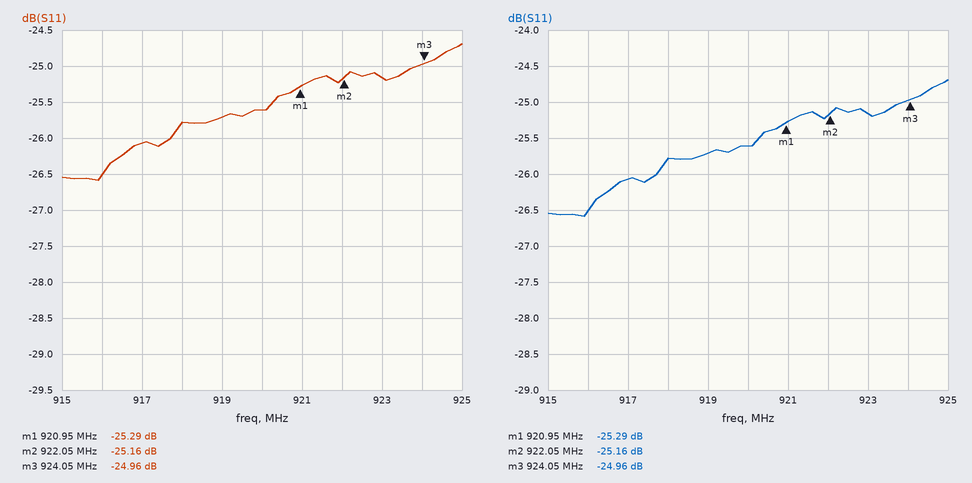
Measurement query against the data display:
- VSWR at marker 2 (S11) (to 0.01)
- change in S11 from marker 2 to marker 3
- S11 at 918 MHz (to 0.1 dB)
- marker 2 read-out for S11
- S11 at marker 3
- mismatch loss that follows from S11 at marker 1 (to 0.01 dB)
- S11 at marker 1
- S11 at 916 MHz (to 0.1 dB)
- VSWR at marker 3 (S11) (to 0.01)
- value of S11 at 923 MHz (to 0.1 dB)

1.12
0.20 dB
-25.8 dB
-25.16 dB
-24.96 dB
0.01 dB
-25.29 dB
-26.5 dB
1.12
-25.2 dB
